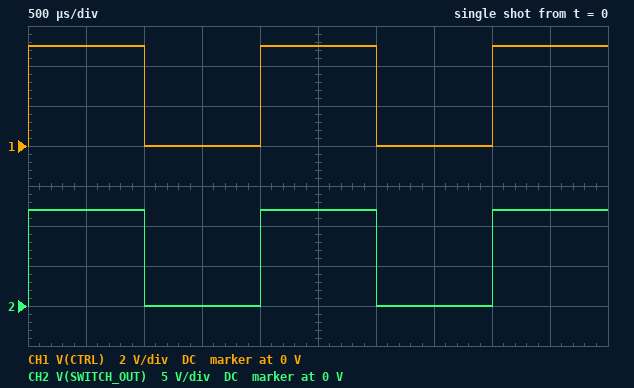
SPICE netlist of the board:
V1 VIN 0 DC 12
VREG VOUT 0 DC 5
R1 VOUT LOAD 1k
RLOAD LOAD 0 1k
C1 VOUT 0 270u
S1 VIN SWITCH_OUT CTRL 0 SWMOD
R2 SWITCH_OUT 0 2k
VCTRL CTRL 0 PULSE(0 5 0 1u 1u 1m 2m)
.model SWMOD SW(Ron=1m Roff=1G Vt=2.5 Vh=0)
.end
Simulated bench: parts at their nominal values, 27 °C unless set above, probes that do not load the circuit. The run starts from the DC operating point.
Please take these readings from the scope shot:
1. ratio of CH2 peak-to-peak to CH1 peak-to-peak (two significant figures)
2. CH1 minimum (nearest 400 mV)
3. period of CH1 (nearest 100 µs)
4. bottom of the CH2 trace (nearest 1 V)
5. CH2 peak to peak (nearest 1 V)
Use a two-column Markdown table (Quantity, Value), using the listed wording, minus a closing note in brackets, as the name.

| Quantity | Value |
|---|---|
| ratio of CH2 peak-to-peak to CH1 peak-to-peak | 2.4 |
| CH1 minimum | 0 V |
| period of CH1 | 2.0 ms |
| bottom of the CH2 trace | 0 V |
| CH2 peak to peak | 12 V |
